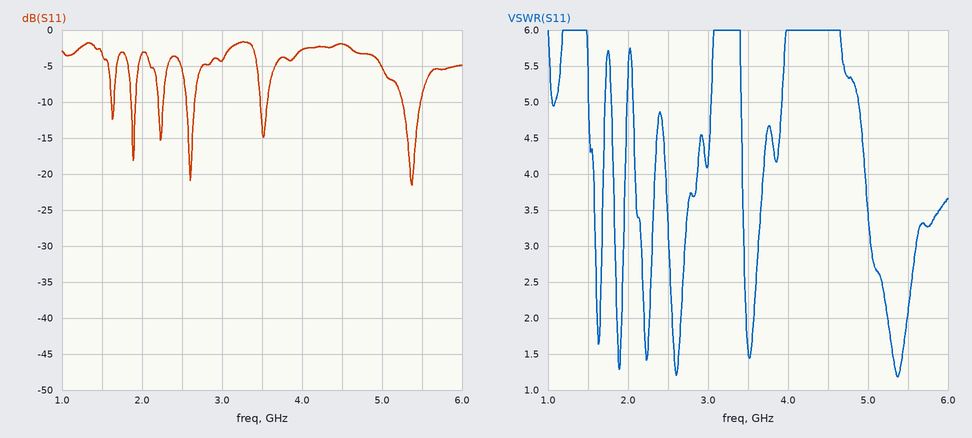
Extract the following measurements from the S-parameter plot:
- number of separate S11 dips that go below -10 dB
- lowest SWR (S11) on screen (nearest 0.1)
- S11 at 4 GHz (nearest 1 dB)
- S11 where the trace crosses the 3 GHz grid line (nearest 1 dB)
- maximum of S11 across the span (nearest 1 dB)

6
1.2
-3 dB
-4 dB
-2 dB
